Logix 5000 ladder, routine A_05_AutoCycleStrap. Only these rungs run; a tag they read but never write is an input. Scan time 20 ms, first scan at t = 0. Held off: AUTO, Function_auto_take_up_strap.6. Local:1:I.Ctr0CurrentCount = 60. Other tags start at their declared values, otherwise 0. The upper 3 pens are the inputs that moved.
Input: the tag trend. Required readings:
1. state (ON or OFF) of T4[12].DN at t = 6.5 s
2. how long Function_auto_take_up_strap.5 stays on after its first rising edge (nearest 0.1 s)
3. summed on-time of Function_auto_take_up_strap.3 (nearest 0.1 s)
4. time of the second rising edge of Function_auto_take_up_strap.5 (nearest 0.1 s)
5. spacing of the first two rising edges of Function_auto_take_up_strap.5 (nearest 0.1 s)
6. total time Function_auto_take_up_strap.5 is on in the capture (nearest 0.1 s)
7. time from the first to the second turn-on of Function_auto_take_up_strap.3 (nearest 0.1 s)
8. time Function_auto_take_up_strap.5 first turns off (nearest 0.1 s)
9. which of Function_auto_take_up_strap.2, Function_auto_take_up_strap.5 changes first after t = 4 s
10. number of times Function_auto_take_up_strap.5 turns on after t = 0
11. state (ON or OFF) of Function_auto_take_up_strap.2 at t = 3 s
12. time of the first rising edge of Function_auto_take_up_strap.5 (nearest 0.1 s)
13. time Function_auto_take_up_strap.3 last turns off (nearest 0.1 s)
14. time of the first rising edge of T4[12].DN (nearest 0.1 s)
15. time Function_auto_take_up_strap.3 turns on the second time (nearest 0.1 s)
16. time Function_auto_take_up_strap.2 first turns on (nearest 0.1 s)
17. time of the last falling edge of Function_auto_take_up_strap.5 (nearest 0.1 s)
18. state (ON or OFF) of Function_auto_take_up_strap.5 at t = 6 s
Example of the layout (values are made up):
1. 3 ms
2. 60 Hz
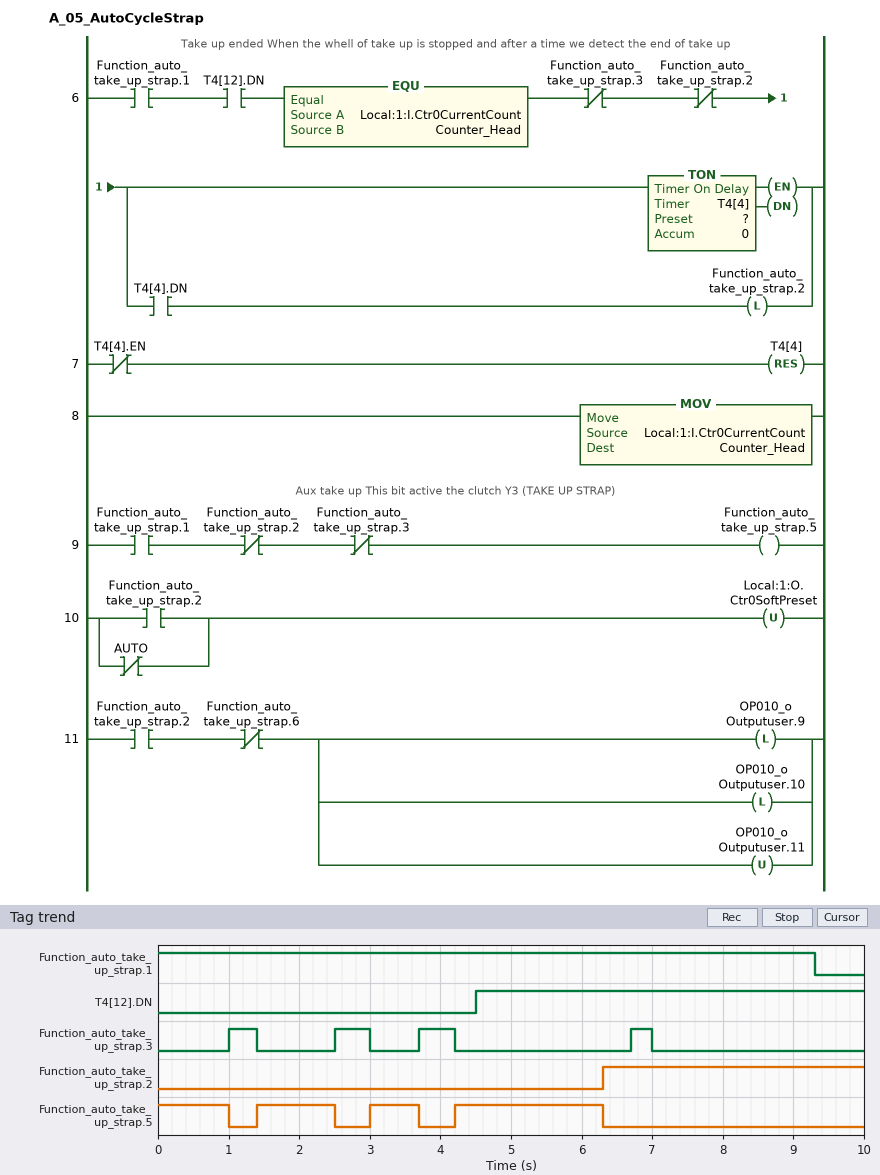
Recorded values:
1. ON
2. 1.1 s
3. 1.7 s
4. 3.0 s
5. 1.6 s
6. 4.9 s
7. 1.5 s
8. 1.0 s
9. Function_auto_take_up_strap.5
10. 3
11. OFF
12. 1.4 s
13. 7.0 s
14. 4.5 s
15. 2.5 s
16. 6.3 s
17. 6.3 s
18. ON
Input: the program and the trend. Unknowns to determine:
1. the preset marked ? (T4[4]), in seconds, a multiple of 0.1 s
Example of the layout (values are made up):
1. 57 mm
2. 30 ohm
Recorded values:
1. 1.8 s
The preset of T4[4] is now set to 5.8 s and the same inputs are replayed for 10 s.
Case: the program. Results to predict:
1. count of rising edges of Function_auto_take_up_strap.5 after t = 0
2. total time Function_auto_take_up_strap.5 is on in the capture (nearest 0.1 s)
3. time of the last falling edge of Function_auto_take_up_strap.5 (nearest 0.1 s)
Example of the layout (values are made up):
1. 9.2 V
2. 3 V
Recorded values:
1. 4
2. 7.6 s
3. 9.3 s
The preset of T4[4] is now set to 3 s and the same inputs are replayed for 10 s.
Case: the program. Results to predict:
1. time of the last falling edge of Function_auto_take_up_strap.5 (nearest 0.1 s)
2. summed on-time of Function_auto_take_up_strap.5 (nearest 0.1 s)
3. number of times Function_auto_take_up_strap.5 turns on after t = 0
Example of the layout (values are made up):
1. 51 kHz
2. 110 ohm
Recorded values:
1. 9.3 s
2. 7.6 s
3. 4
